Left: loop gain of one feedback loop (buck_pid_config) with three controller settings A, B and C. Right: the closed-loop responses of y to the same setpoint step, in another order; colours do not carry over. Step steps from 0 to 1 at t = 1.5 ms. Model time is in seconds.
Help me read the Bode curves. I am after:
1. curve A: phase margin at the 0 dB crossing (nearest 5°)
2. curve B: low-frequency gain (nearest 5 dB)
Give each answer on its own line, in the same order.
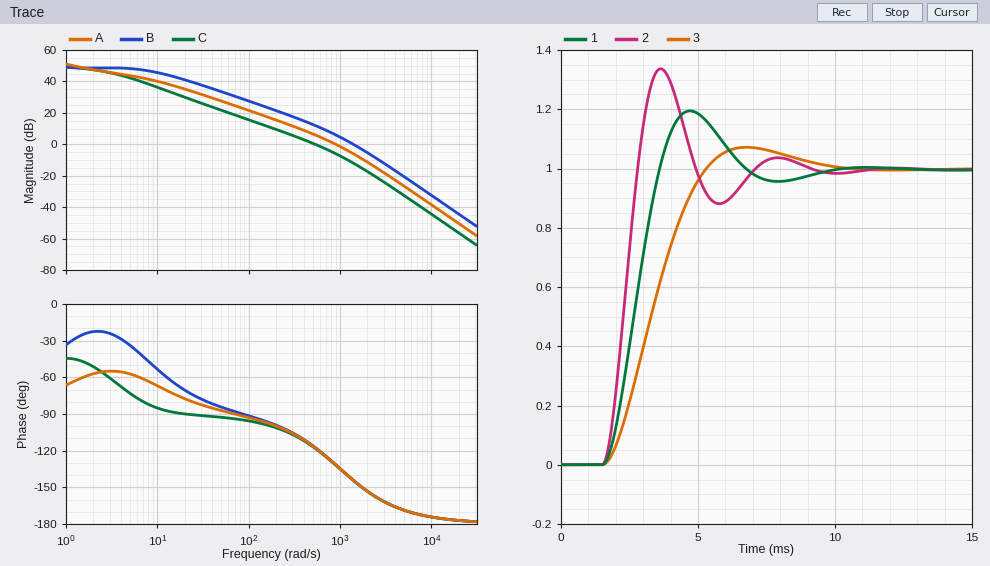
50°
50 dB
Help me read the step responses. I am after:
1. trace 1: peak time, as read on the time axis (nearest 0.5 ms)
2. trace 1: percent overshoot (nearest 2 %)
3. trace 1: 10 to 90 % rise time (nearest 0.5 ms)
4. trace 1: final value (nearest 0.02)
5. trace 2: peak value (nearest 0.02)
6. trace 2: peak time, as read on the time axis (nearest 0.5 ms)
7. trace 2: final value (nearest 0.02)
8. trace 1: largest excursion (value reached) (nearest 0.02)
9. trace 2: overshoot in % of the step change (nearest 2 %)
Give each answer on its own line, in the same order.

4.5 ms
20 %
1.5 ms
1.00
1.34
3.5 ms
1.00
1.20
34 %
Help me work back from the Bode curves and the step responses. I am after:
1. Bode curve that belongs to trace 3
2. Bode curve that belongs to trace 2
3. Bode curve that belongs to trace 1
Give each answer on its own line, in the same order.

C
B
A
